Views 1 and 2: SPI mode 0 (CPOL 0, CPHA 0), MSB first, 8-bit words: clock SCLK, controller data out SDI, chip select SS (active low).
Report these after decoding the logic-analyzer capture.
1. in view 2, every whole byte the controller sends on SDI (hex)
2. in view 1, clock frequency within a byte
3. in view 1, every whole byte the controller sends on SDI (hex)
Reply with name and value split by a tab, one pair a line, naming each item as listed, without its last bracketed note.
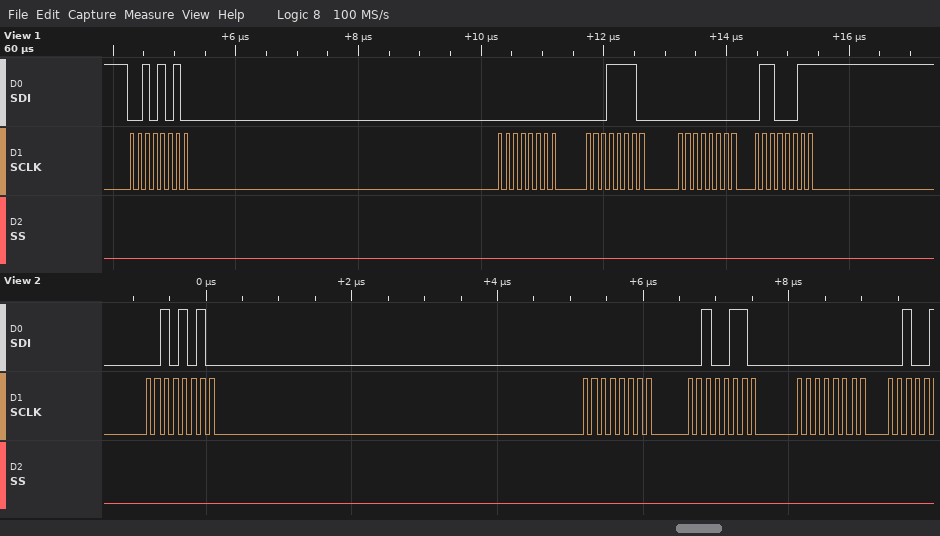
in view 2, every whole byte the controller sends on SDI	2A 00 26 00
in view 1, clock frequency within a byte	8 MHz
in view 1, every whole byte the controller sends on SDI	2A 00 1E 00 63
